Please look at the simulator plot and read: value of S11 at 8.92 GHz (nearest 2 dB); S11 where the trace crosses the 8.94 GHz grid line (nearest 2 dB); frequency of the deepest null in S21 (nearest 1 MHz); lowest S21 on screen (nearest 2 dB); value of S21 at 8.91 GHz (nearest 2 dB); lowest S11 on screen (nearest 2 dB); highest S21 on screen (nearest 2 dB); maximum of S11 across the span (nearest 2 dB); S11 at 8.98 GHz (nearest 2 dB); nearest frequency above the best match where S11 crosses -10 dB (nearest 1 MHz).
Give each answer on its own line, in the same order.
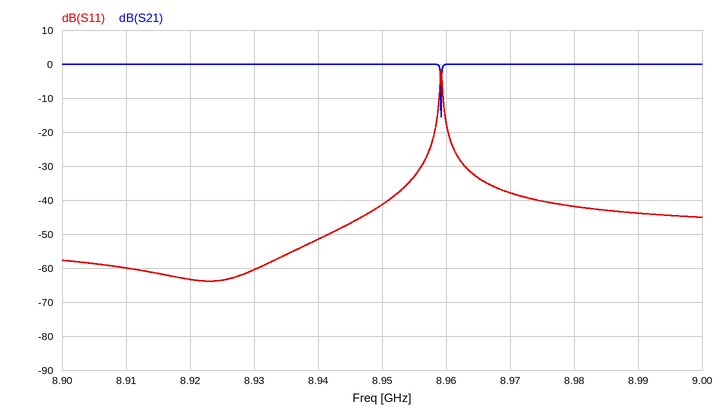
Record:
-64 dB
-52 dB
8.959 GHz
-16 dB
0 dB
-64 dB
0 dB
-2 dB
-42 dB
8.959 GHz
